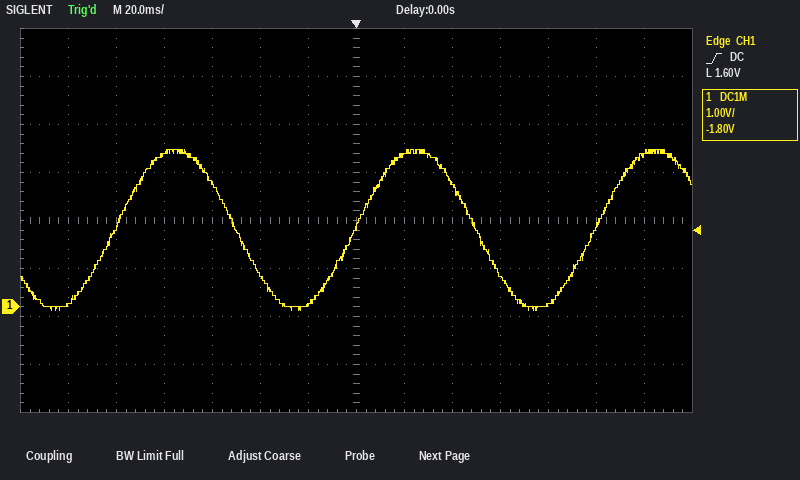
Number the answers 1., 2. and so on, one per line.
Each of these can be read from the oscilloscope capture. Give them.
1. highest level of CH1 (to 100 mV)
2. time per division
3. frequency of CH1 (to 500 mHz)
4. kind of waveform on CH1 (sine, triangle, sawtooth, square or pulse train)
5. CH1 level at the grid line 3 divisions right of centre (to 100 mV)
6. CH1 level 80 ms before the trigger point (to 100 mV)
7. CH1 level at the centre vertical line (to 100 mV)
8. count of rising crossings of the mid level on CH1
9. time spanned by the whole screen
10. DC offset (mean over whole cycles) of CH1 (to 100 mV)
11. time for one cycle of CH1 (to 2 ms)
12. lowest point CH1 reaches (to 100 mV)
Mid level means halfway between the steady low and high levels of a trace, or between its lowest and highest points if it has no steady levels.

1. 3.3 V
2. 20 ms
3. 10.0 Hz
4. sine
5. 700 mV
6. 3.2 V
7. 1.7 V
8. 3
9. 280 ms
10. 1.6 V
11. 100 ms
12. -100 mV
